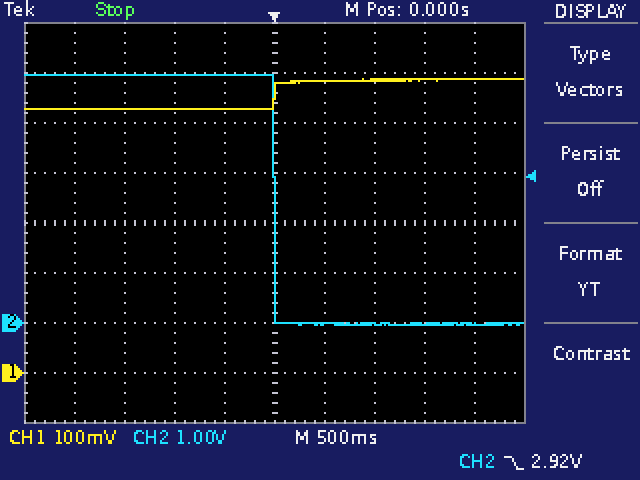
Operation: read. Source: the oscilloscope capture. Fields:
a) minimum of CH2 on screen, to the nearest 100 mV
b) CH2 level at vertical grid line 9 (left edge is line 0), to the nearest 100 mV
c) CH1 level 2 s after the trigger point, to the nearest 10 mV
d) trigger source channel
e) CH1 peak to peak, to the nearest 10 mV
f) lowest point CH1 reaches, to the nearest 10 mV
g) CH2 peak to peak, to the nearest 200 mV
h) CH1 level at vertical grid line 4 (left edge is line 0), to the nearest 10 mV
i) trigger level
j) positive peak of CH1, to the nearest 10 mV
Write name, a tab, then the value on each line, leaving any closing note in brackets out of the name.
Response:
minimum of CH2 on screen, to the nearest 100 mV	0.0 V
CH2 level at vertical grid line 9 (left edge is line 0), to the nearest 100 mV	0.0 V
CH1 level 2 s after the trigger point, to the nearest 10 mV	590 mV
trigger source channel	CH2
CH1 peak to peak, to the nearest 10 mV	60 mV
lowest point CH1 reaches, to the nearest 10 mV	530 mV
CH2 peak to peak, to the nearest 200 mV	5.0 V
CH1 level at vertical grid line 4 (left edge is line 0), to the nearest 10 mV	530 mV
trigger level	2.92 V
positive peak of CH1, to the nearest 10 mV	590 mV
